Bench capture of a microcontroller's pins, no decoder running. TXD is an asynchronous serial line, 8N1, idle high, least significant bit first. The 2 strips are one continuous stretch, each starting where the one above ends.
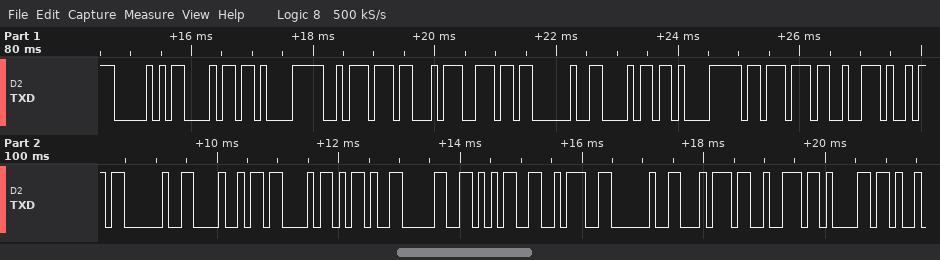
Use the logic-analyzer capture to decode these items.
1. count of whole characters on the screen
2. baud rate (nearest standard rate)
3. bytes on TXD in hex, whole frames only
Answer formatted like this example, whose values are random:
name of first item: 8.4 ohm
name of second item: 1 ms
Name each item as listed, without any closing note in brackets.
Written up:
count of whole characters on the screen: 23
baud rate: 9600 baud
bytes on TXD in hex, whole frames only: 50 68 E1 BA A3 6E 20 68 E1 BB 93 69 20 48 43 2D 30 35 3A 20 74 72 61
